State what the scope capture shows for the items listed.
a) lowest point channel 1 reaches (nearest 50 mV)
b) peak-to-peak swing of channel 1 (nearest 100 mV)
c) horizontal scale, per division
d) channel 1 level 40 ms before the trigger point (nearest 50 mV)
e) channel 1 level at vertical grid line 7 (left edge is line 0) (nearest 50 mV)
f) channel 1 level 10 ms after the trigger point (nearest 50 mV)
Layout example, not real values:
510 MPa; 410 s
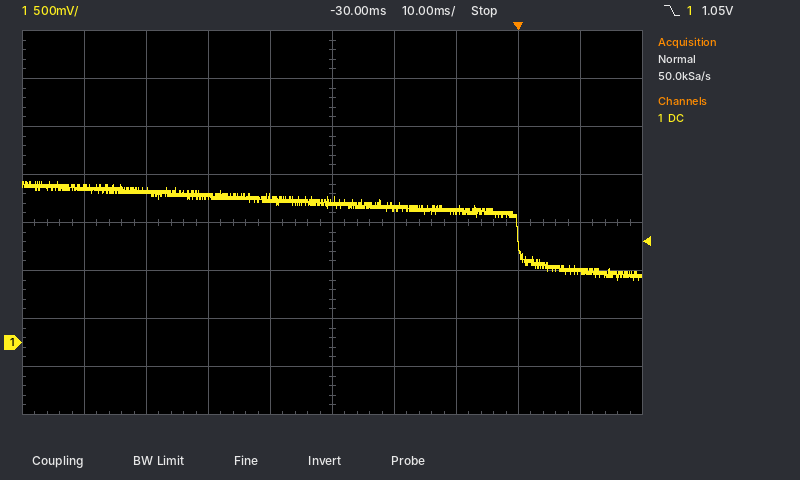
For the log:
650 mV; 1.00 V; 10 ms; 1.50 V; 1.35 V; 750 mV
